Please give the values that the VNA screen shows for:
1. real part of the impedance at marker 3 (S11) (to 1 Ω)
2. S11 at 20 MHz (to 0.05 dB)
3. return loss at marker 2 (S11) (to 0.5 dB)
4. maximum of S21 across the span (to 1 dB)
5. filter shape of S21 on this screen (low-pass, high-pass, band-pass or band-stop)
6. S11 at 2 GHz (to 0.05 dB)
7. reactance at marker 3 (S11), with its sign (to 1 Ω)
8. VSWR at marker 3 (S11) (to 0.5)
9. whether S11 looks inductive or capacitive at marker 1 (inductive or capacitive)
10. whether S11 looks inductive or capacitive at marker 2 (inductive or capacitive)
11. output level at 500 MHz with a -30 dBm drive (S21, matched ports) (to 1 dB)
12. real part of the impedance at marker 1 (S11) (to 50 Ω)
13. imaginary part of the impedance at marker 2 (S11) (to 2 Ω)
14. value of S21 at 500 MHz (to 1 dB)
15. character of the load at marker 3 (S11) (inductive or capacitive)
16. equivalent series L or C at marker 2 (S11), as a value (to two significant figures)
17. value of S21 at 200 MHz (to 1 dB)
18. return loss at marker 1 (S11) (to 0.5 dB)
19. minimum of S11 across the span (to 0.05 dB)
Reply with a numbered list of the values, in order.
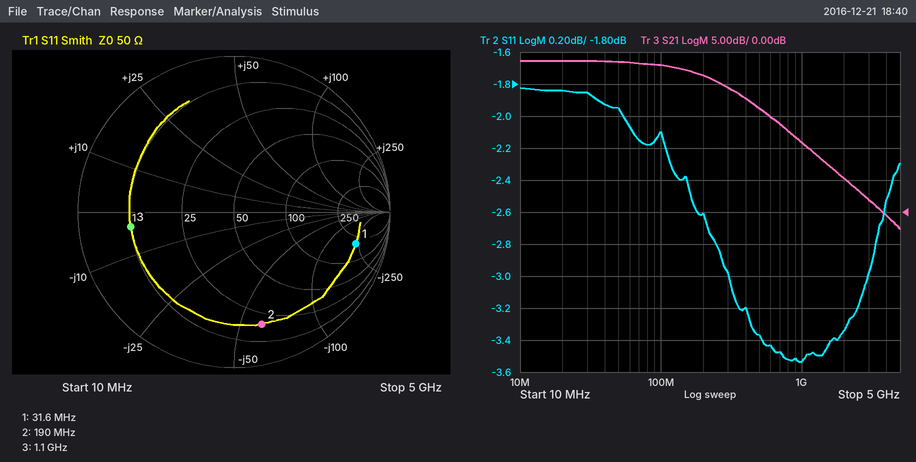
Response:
1. 10 Ω
2. -1.85 dB
3. 2.5 dB
4. 24 dB
5. low-pass
6. -3.35 dB
7. -3 Ω
8. 5.0
9. capacitive
10. capacitive
11. -14 dBm
12. 200 Ω
13. -60 Ω
14. 16 dB
15. capacitive
16. 14 pF
17. 21 dB
18. 2.0 dB
19. -3.55 dB
